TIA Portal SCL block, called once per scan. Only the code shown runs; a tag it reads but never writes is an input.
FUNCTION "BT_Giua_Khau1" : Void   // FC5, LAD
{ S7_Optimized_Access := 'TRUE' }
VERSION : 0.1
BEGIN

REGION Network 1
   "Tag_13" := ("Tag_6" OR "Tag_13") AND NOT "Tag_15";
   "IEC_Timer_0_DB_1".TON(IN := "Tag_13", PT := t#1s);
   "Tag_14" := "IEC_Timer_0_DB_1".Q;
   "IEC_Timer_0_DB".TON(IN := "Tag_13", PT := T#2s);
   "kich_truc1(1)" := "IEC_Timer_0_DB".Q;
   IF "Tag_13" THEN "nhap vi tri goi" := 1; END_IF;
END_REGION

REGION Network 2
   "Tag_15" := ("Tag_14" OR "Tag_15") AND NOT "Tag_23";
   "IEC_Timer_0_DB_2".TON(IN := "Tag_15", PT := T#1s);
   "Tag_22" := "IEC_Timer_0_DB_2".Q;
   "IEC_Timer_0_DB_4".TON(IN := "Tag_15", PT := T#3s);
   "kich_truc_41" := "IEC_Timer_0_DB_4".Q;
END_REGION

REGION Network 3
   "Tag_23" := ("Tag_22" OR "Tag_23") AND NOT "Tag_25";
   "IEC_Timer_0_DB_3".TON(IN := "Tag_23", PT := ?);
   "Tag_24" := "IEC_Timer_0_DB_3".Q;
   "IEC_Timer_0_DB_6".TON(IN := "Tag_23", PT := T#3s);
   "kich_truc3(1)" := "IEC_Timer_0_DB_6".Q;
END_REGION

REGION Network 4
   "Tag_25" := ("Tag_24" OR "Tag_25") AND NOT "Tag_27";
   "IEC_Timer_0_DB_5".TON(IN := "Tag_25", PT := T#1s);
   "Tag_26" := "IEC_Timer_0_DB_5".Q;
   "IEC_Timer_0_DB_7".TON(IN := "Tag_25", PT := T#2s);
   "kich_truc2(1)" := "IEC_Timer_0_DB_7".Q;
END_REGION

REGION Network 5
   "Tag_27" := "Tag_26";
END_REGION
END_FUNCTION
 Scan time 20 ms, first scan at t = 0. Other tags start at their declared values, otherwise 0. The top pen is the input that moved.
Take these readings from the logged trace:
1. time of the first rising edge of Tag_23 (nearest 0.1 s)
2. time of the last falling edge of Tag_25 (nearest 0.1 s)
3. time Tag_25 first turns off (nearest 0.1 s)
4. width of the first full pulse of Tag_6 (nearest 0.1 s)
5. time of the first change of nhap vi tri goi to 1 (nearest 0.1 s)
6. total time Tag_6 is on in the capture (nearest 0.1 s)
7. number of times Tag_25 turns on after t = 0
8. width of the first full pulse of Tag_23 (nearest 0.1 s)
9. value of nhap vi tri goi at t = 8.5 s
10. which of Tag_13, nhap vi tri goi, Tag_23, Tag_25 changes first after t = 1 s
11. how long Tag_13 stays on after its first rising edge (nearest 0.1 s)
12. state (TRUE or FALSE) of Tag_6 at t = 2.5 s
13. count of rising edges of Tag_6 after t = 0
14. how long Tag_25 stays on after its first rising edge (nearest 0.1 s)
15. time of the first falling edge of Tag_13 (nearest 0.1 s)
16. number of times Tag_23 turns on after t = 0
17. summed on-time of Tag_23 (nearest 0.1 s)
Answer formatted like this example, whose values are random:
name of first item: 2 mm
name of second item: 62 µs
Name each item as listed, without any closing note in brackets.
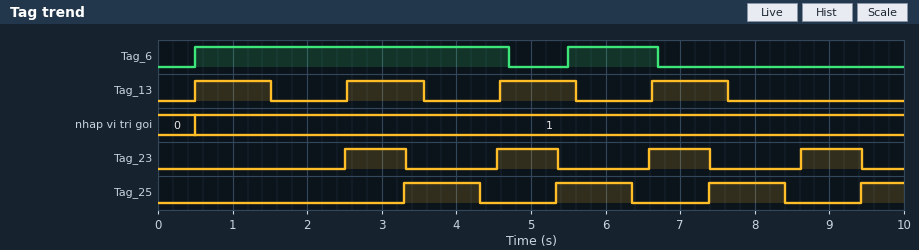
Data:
time of the first rising edge of Tag_23: 2.5 s
time of the last falling edge of Tag_25: 8.4 s
time Tag_25 first turns off: 4.3 s
width of the first full pulse of Tag_6: 4.2 s
time of the first change of nhap vi tri goi to 1: 0.5 s
total time Tag_6 is on in the capture: 5.4 s
number of times Tag_25 turns on after t = 0: 4
width of the first full pulse of Tag_23: 0.8 s
value of nhap vi tri goi at t = 8.5 s: 1
which of Tag_13, nhap vi tri goi, Tag_23, Tag_25 changes first after t = 1 s: Tag_13
how long Tag_13 stays on after its first rising edge: 1.0 s
state (TRUE or FALSE) of Tag_6 at t = 2.5 s: TRUE
count of rising edges of Tag_6 after t = 0: 2
how long Tag_25 stays on after its first rising edge: 1.0 s
time of the first falling edge of Tag_13: 1.5 s
number of times Tag_23 turns on after t = 0: 4
summed on-time of Tag_23: 3.3 s
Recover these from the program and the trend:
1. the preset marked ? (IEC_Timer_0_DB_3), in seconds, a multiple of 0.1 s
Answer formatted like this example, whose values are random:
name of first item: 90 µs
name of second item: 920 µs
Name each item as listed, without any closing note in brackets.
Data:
the preset marked ? (IEC_Timer_0_DB_3), in seconds, a multiple of 0.1 s: 0.8 s
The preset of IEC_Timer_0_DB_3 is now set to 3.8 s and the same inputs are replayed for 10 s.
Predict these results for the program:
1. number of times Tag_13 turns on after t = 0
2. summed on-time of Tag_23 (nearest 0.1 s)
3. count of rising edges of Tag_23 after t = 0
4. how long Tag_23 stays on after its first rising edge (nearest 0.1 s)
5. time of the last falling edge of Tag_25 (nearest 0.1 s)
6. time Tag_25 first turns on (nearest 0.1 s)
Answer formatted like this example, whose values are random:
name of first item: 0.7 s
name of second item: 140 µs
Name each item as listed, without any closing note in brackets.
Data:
number of times Tag_13 turns on after t = 0: 2
summed on-time of Tag_23: 6.5 s
count of rising edges of Tag_23 after t = 0: 2
how long Tag_23 stays on after its first rising edge: 3.8 s
time of the last falling edge of Tag_25: 7.3 s
time Tag_25 first turns on: 6.3 s
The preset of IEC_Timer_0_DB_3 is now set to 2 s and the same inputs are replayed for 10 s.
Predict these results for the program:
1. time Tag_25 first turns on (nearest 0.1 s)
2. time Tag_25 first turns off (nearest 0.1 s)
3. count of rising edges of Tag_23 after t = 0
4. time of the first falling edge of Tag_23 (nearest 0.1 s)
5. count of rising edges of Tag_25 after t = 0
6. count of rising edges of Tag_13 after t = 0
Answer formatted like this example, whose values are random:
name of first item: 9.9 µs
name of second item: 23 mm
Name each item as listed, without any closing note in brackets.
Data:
time Tag_25 first turns on: 4.5 s
time Tag_25 first turns off: 5.5 s
count of rising edges of Tag_23 after t = 0: 3
time of the first falling edge of Tag_23: 4.5 s
count of rising edges of Tag_25 after t = 0: 2
count of rising edges of Tag_13 after t = 0: 3
